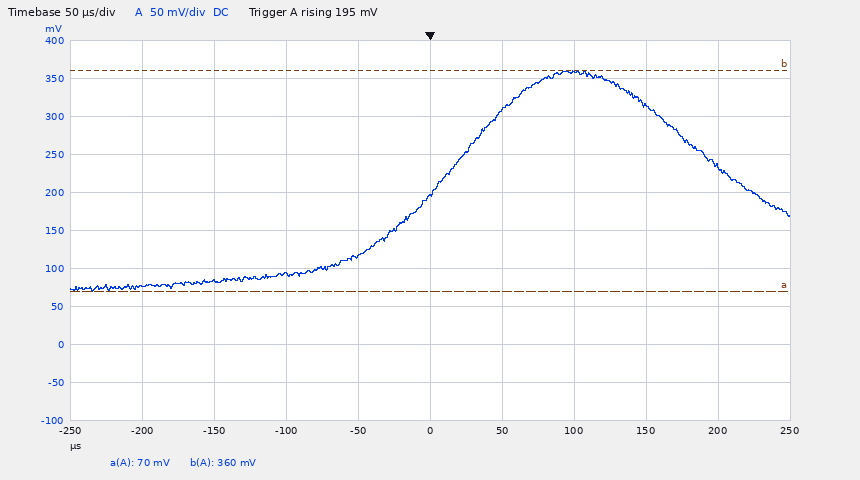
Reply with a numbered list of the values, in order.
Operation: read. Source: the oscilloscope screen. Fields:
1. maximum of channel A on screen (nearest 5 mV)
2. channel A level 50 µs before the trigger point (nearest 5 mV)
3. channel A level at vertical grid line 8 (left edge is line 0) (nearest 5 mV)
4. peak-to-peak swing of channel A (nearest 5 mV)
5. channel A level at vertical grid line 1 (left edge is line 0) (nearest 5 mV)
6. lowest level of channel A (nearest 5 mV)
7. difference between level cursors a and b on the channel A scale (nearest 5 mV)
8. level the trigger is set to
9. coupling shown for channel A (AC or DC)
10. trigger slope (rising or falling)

1. 360 mV
2. 115 mV
3. 315 mV
4. 290 mV
5. 75 mV
6. 70 mV
7. 290 mV
8. 195 mV
9. DC
10. rising
